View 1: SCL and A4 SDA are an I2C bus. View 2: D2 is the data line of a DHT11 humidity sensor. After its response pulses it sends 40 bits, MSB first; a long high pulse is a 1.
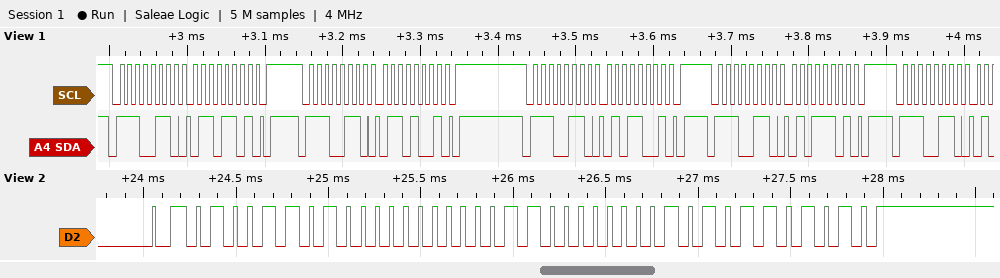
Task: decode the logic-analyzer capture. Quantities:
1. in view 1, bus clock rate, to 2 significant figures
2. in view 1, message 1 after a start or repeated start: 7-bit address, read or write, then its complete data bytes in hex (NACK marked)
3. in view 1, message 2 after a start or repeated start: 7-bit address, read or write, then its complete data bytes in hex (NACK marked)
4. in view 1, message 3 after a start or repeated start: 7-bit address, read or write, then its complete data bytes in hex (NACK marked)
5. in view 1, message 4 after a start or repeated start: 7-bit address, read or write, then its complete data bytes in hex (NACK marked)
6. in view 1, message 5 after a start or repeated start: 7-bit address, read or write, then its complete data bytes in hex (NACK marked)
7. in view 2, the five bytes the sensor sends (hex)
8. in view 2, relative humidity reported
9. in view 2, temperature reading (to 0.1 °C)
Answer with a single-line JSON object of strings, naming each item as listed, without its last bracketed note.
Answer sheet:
{"in view 1, bus clock rate, to 2 significant figures": "100 kHz", "in view 1, message 1 after a start or repeated start: 7-bit address, read or write, then its complete data bytes in hex": "0x73 write: 6D", "in view 1, message 2 after a start or repeated start: 7-bit address, read or write, then its complete data bytes in hex": "0x73 write: 69", "in view 1, message 3 after a start or repeated start: 7-bit address, read or write, then its complete data bytes in hex": "0x73 write: 59", "in view 1, message 4 after a start or repeated start: 7-bit address, read or write, then its complete data bytes in hex": "0x73 write: 5D", "in view 1, message 5 after a start or repeated start: 7-bit address, read or write, then its complete data bytes in hex": "0x73 write", "in view 2, the five bytes the sensor sends": "4D 00 18 05 6A", "in view 2, relative humidity reported": "77 %", "in view 2, temperature reading": "24.5 °C"}
